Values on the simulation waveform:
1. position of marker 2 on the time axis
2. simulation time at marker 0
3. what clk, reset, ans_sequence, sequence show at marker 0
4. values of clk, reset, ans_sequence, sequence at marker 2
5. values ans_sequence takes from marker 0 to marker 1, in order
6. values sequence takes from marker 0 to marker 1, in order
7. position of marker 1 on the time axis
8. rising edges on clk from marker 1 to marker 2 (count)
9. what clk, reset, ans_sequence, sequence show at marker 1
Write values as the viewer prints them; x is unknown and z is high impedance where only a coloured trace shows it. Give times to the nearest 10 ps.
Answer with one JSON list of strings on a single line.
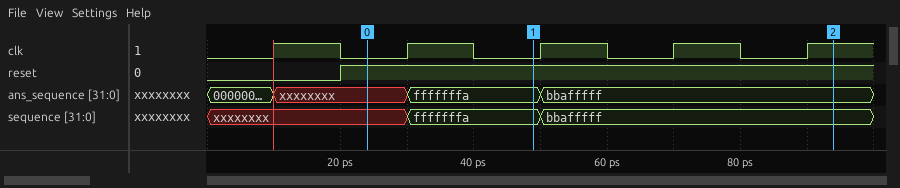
["90 ps", "20 ps", "clk=0, reset=1, ans_sequence=xxxxxxxx, sequence=xxxxxxxx", "clk=1, reset=1, ans_sequence=bbafffff, sequence=bbafffff", "xxxxxxxx, fffffffa", "xxxxxxxx, fffffffa", "50 ps", "3", "clk=0, reset=1, ans_sequence=fffffffa, sequence=fffffffa"]
